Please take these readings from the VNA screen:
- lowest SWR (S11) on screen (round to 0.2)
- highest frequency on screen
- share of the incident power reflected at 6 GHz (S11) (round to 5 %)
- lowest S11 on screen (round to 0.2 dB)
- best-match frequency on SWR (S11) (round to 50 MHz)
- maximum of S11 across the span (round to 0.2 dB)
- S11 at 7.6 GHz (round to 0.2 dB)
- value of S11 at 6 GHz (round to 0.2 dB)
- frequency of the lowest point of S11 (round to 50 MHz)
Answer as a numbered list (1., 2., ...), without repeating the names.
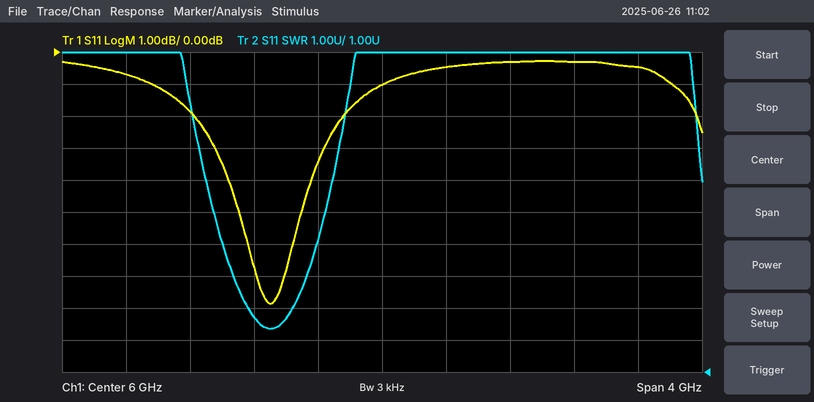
1. 2.4
2. 8 GHz
3. 80 %
4. -7.8 dB
5. 5.30 GHz
6. -0.2 dB
7. -0.4 dB
8. -1.0 dB
9. 5.30 GHz
